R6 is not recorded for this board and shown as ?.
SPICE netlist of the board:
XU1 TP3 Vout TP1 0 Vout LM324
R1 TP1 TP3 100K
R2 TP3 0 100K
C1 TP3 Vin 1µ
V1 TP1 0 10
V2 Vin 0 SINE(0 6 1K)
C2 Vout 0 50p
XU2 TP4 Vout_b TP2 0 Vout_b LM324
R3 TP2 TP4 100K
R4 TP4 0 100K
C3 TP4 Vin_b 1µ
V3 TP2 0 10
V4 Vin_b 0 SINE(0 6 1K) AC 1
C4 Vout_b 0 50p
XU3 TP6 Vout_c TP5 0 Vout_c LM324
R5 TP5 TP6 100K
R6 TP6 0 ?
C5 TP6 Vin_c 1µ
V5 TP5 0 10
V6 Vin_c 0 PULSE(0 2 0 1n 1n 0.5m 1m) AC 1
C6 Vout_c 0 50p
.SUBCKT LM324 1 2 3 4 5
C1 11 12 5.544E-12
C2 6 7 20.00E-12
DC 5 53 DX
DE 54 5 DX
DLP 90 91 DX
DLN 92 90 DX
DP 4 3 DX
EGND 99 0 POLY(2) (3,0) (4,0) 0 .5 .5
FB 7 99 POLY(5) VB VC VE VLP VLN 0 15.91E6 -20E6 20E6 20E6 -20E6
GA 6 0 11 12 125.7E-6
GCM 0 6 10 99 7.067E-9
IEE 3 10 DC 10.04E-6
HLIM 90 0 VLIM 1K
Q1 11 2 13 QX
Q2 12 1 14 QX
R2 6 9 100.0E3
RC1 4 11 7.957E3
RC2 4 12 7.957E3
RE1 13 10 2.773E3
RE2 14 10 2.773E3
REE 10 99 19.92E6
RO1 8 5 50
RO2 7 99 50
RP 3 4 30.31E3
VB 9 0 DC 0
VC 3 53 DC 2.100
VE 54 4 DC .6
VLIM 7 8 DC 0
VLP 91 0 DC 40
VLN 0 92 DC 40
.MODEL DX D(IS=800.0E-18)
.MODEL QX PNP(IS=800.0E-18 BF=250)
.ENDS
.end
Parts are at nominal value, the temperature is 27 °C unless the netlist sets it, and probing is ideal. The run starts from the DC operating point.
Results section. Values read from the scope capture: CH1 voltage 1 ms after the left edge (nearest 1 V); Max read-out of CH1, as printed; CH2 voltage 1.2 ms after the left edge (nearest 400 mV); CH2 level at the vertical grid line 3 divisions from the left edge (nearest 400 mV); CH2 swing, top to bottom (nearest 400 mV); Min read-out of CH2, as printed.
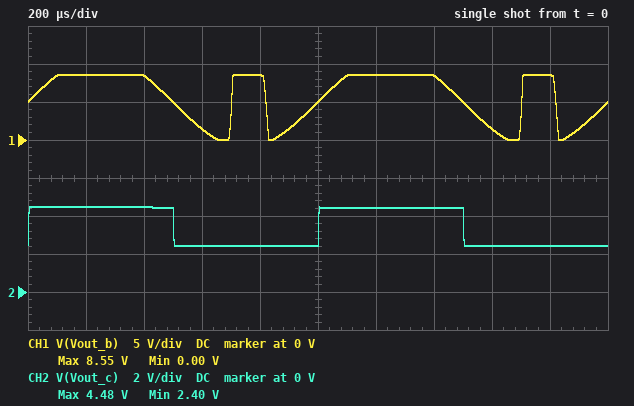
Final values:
5 V
8.55 V
4.4 V
2.4 V
2.0 V
2.40 V
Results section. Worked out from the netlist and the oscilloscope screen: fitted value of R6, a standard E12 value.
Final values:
33 kΩ
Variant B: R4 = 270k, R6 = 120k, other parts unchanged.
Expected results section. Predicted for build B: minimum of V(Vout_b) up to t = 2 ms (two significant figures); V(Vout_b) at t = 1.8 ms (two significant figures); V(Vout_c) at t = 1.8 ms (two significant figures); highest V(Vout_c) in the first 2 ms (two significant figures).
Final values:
1.3 V
1.6 V
5.4 V
7.5 V
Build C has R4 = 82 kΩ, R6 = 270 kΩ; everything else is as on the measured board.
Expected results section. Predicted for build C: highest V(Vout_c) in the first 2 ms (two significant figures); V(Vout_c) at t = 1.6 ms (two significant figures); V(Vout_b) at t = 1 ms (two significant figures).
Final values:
8.5 V
7.3 V
4.5 V
